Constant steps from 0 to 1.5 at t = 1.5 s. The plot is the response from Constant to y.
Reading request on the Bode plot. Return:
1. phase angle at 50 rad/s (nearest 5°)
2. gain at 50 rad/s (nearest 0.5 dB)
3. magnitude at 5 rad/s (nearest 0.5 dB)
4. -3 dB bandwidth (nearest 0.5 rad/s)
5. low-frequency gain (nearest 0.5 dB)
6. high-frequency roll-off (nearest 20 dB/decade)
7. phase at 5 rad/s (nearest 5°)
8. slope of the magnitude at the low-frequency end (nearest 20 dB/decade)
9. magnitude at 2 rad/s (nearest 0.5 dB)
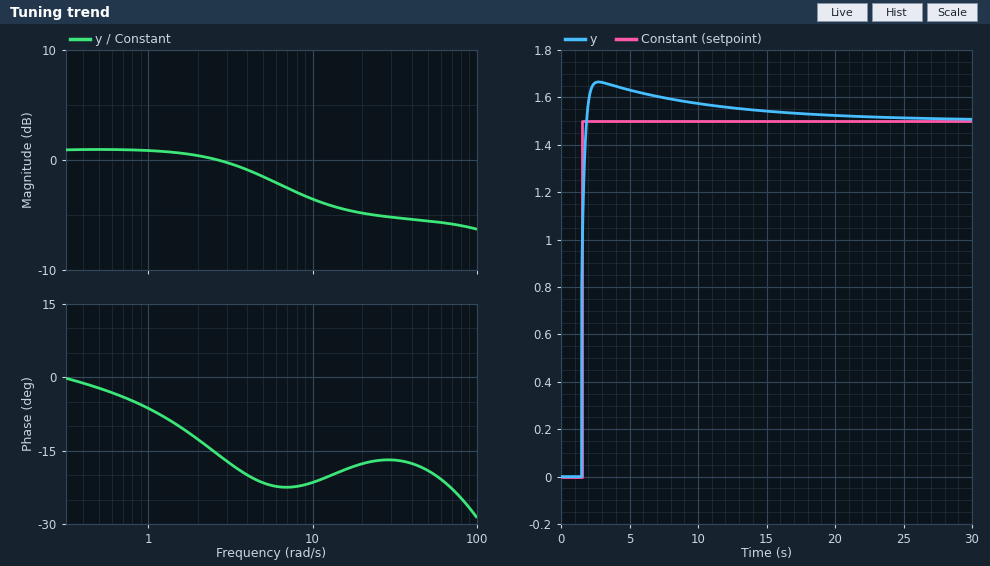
-20°
-5.5 dB
-1.5 dB
6.0 rad/s
1.0 dB
0 dB/decade
-20°
0 dB/decade
0.5 dB
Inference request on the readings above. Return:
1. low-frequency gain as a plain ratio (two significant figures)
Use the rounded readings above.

1.1
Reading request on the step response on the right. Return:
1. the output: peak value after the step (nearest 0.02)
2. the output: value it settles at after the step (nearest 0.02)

1.66
1.50
